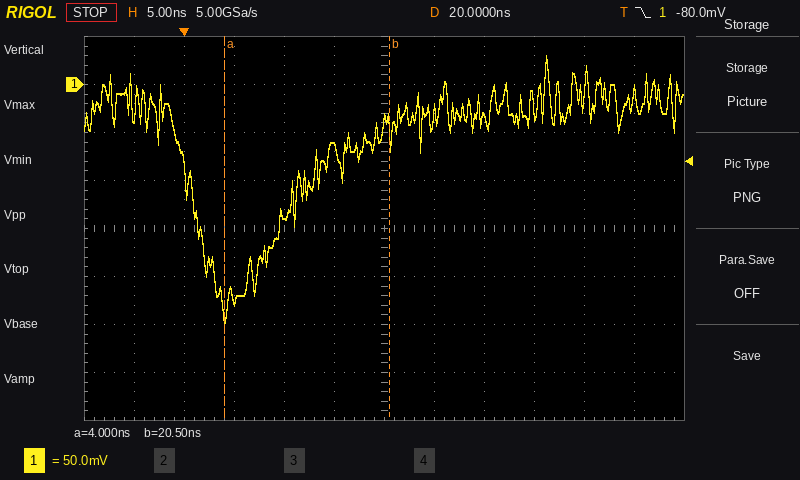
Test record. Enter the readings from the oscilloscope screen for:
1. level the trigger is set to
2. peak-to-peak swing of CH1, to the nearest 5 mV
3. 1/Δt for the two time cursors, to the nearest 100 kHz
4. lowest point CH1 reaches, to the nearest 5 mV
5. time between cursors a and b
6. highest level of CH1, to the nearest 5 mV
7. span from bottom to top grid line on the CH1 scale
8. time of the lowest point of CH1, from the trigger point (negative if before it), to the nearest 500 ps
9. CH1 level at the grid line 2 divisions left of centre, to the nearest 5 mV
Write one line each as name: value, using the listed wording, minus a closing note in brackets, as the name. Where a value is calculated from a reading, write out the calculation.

level the trigger is set to: -80.0 mV
peak-to-peak swing of CH1, to the nearest 5 mV: 30 mV − (-250 mV) = 280 mV
1/Δt for the two time cursors, to the nearest 100 kHz: 1 / 16.5 ns ≈ 60.6 MHz
lowest point CH1 reaches, to the nearest 5 mV: -250 mV
time between cursors a and b: 20.5 ns − (4 ns) = 16.5 ns
highest level of CH1, to the nearest 5 mV: 30 mV
span from bottom to top grid line on the CH1 scale: 400 mV
time of the lowest point of CH1, from the trigger point (negative if before it), to the nearest 500 ps: +4.0 ns
CH1 level at the grid line 2 divisions left of centre, to the nearest 5 mV: -135 mV
